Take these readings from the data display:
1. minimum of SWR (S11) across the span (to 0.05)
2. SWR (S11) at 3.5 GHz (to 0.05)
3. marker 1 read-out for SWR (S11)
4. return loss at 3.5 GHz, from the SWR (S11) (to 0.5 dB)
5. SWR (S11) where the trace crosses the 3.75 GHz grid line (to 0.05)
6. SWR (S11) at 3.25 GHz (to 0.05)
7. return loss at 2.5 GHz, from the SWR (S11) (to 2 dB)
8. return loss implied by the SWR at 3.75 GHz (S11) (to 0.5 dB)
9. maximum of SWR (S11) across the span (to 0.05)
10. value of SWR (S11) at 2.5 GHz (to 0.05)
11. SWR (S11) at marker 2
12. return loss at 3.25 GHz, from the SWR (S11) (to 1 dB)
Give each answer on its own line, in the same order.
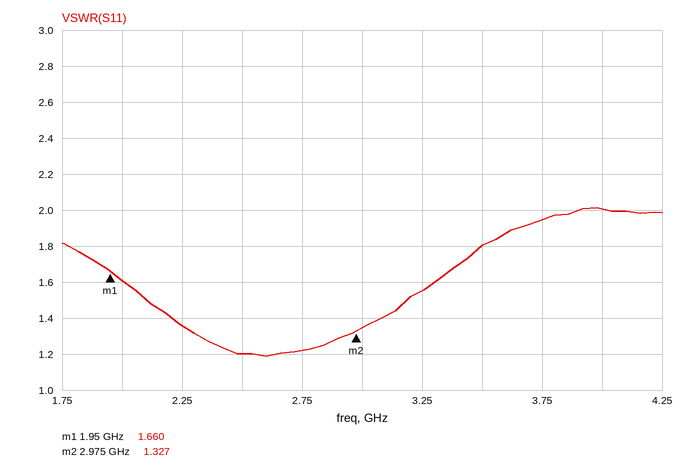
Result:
1.20
1.80
1.660
11.0 dB
1.95
1.55
20 dB
10.0 dB
2.00
1.20
1.327
13 dB
